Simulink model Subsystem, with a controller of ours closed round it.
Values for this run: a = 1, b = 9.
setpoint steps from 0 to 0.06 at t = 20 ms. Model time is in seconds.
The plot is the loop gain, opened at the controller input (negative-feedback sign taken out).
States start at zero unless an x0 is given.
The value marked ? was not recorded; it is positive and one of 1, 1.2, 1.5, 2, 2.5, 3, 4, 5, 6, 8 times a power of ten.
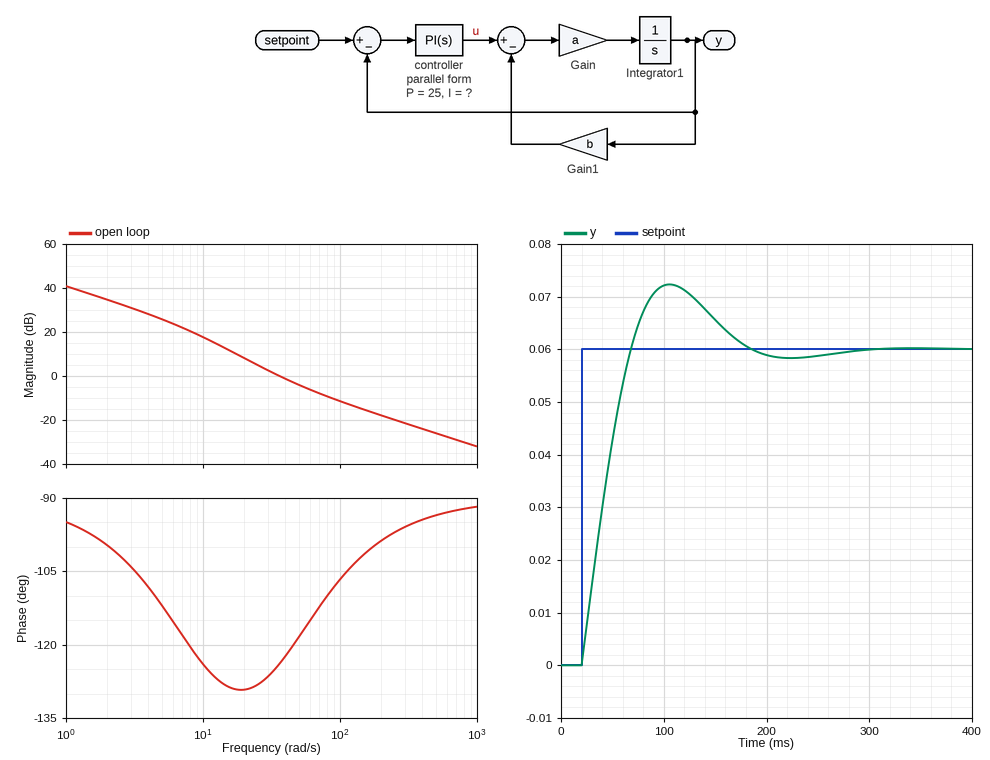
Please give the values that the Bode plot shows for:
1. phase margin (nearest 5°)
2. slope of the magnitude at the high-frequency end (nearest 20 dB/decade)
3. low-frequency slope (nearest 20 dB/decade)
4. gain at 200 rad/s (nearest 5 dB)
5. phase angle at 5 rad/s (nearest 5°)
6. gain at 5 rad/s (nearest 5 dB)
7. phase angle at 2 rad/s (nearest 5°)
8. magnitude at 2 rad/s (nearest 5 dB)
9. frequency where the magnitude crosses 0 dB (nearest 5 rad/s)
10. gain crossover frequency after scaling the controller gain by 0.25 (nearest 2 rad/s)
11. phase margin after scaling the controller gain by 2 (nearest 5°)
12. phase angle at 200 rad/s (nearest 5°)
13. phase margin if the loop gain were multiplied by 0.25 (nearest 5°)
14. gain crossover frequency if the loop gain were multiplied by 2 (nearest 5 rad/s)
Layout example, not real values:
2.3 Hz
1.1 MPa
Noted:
55°
-20 dB/decade
-20 dB/decade
-20 dB
-110°
25 dB
-100°
35 dB
35 rad/s
16 rad/s
65°
-100°
50°
60 rad/s
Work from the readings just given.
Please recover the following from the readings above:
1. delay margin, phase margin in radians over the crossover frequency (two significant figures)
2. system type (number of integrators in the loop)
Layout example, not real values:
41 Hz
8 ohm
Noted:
0.027 s
1
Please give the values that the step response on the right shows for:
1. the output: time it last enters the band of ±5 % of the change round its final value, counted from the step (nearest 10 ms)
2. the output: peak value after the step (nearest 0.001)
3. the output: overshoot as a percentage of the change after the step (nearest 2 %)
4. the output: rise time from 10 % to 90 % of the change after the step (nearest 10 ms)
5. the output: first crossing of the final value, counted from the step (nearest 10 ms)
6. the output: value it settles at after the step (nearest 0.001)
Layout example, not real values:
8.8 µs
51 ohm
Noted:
140 ms
0.072
20 %
40 ms
50 ms
0.060
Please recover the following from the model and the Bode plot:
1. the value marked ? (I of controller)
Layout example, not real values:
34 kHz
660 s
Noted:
1000
